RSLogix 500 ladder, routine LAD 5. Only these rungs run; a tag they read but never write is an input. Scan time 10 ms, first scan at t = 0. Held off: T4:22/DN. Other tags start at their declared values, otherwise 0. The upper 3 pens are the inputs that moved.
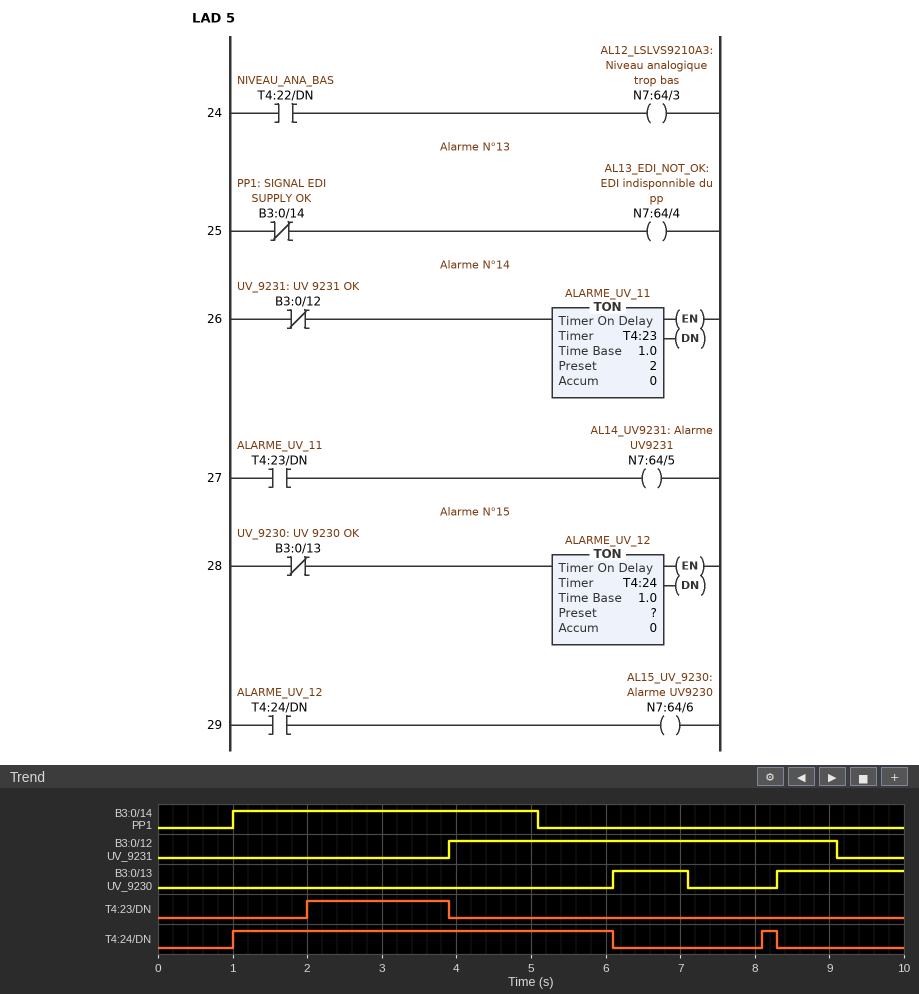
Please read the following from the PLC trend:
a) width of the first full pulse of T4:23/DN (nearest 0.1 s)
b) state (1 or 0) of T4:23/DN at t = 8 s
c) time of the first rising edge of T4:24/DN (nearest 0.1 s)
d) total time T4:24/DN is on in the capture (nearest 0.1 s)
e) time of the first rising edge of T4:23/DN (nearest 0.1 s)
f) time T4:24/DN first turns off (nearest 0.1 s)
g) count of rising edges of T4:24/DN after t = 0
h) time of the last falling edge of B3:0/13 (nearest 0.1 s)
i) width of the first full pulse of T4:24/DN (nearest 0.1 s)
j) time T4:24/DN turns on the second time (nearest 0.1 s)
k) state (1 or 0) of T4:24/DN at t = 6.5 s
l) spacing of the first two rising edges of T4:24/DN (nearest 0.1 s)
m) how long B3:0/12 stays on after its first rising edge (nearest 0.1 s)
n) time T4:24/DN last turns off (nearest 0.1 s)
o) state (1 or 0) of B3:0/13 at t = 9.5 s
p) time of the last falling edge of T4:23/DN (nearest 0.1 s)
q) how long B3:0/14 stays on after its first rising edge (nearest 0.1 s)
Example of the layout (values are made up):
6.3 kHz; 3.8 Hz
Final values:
1.9 s; 0; 1.0 s; 5.3 s; 2.0 s; 6.1 s; 2; 7.1 s; 5.1 s; 8.1 s; 0; 7.1 s; 5.2 s; 8.3 s; 1; 3.9 s; 4.1 s
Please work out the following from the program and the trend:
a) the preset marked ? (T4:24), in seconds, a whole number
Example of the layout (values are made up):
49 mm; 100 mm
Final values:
1 s
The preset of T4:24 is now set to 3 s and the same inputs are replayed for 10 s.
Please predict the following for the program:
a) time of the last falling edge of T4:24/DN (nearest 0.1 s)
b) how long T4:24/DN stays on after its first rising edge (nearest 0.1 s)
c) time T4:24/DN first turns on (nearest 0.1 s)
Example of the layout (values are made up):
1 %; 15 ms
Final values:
6.1 s; 3.1 s; 3.0 s
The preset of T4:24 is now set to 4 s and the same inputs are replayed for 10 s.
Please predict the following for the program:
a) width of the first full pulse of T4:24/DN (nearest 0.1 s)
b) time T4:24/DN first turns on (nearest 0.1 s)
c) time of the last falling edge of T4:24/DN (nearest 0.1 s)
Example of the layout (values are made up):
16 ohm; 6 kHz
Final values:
2.1 s; 4.0 s; 6.1 s
